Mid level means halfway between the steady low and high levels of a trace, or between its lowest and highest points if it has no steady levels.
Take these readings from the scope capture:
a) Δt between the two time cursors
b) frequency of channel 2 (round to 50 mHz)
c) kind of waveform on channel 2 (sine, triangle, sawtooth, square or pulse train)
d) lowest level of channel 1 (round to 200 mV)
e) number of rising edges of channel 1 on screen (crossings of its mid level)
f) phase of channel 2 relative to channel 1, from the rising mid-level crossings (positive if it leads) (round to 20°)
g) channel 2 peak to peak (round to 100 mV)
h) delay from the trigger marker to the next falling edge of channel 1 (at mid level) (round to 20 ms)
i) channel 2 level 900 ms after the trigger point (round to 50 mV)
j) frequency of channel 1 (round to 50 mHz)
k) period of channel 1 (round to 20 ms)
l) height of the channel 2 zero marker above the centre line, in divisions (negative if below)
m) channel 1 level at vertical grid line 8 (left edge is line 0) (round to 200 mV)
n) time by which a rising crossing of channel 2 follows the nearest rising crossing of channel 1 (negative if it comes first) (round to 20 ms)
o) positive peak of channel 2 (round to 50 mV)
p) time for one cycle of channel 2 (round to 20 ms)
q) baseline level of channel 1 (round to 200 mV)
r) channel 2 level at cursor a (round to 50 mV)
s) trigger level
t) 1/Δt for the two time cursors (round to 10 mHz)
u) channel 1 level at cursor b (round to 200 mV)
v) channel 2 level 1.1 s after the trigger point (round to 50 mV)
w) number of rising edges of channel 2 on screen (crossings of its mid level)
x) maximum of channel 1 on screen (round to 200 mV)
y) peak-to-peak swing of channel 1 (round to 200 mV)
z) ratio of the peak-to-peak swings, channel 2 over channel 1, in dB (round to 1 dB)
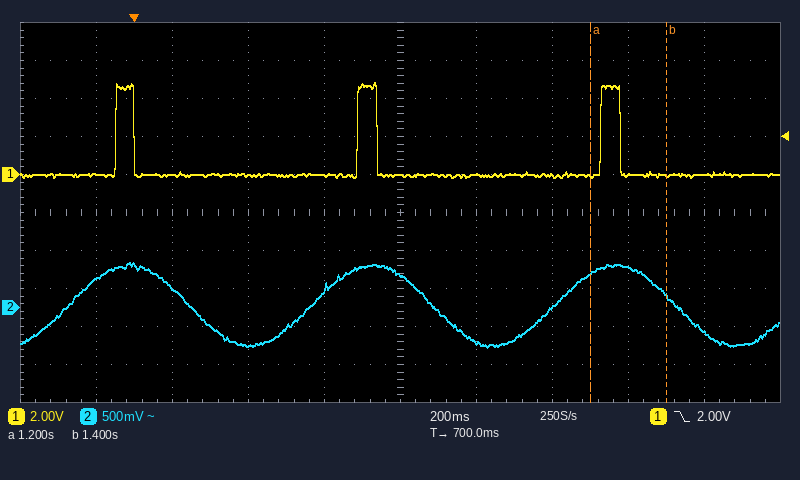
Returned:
200 ms
1.55 Hz
sine
-200 mV
3
+60°
1.10 V
640 ms
-450 mV
1.55 Hz
640 ms
-2.5 div
0.0 V
-120 ms
600 mV
640 ms
0.0 V
450 mV
2.00 V
5.00 Hz
0.0 V
0 mV
3
4.8 V
5.0 V
-13 dB
